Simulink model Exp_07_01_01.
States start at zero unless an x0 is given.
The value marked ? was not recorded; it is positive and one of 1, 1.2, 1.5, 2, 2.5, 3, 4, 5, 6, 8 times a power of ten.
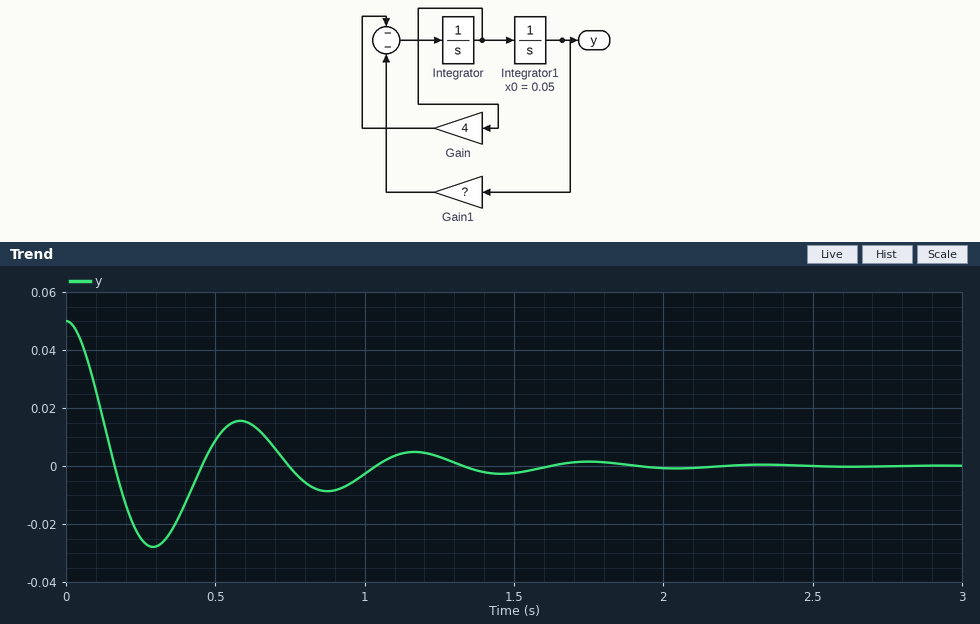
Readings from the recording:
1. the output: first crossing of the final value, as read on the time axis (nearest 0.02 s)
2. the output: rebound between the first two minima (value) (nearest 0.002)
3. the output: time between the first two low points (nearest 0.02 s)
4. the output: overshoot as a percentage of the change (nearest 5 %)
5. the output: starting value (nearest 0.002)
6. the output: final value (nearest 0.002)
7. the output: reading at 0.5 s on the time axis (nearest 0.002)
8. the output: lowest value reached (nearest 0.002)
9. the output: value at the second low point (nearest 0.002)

0.16 s
0.016
0.58 s
55 %
0.050
0.000
0.008
-0.028
-0.008
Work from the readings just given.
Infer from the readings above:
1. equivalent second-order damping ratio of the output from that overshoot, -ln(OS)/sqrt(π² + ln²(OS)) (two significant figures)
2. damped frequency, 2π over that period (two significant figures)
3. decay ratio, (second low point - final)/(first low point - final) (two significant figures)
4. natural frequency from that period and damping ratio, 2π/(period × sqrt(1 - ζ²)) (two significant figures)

0.19
11 rad/s
0.29
11 rad/s
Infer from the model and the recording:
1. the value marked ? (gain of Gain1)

120
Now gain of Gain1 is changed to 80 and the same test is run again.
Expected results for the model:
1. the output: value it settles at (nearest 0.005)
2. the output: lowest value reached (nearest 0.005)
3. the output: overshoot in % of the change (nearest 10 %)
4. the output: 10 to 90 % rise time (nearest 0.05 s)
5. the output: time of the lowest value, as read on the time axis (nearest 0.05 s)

0.000
-0.025
50 %
0.15 s
0.35 s
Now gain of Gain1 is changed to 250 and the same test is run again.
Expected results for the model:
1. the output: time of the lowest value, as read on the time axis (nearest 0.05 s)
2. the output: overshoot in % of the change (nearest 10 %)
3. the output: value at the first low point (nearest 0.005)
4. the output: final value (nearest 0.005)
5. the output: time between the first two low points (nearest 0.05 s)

0.20 s
70 %
-0.035
0.000
0.40 s
